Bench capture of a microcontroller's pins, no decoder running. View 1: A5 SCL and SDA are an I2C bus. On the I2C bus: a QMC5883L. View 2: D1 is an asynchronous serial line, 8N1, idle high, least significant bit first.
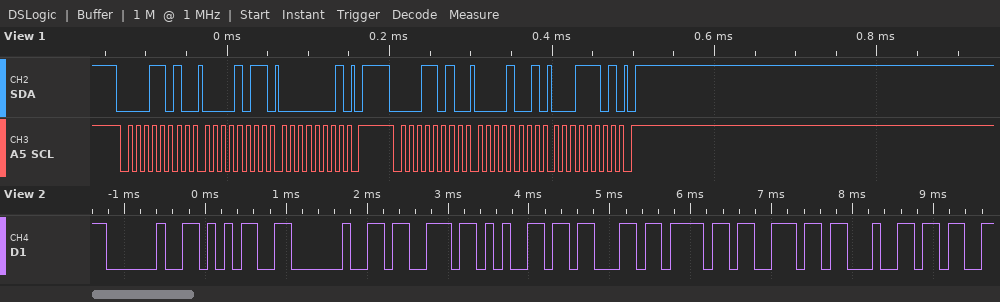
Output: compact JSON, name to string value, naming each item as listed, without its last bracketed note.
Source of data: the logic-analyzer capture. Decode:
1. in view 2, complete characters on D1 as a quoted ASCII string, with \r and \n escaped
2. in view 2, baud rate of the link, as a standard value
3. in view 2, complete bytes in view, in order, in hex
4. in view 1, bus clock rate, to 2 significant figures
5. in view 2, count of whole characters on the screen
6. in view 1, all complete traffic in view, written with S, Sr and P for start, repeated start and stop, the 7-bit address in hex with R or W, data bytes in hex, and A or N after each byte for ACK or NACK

{"in view 2, complete characters on D1 as a quoted ASCII string, with \\r and \\n escaped": "\" 5 second\"", "in view 2, baud rate of the link, as a standard value": "9600 baud", "in view 2, complete bytes in view, in order, in hex": "20 35 20 73 65 63 6F 6E 64", "in view 1, bus clock rate, to 2 significant figures": "100 kHz", "in view 2, count of whole characters on the screen": "9", "in view 1, all complete traffic in view, written with S, Sr and P for start, repeated start and stop, the 7-bit address in hex with R or W, data bytes in hex, and A or N after each byte for ACK or NACK": "S 0DW A 0B A 01 A P S 0DW A 09 A 1D A P"}
